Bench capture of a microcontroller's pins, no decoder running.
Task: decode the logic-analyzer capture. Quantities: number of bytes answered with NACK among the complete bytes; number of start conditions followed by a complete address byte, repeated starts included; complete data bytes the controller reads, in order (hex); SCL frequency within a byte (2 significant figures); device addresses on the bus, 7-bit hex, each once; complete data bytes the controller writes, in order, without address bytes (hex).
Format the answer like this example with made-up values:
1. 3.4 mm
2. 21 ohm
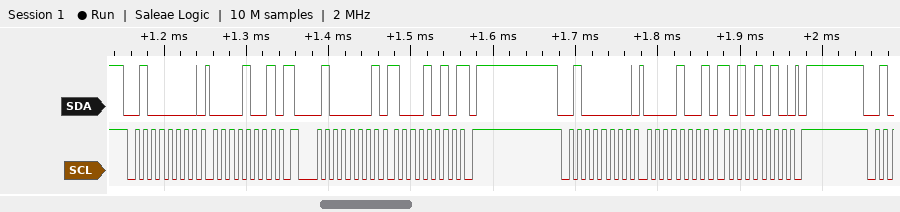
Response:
1. 1
2. 3
3. 8A
4. 100 kHz
5. 0x20
6. 09 09 AA
